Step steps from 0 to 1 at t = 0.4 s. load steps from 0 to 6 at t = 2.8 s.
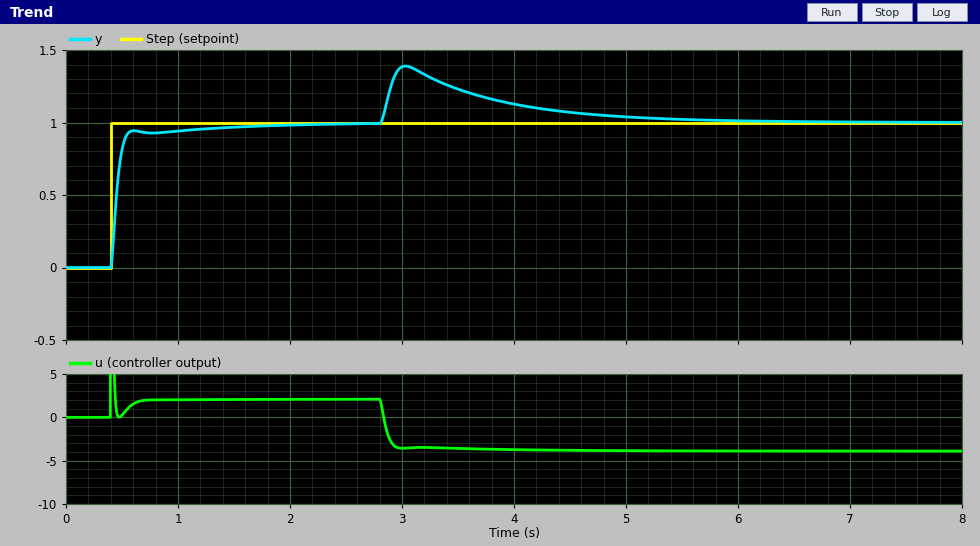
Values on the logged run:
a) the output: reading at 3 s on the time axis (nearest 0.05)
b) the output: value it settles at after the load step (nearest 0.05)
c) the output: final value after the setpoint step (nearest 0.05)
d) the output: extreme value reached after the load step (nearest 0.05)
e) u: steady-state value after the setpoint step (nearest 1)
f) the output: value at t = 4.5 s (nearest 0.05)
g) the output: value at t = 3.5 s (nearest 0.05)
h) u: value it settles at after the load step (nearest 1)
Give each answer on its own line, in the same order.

1.40
1.00
1.00
1.40
2
1.05
1.25
-4
